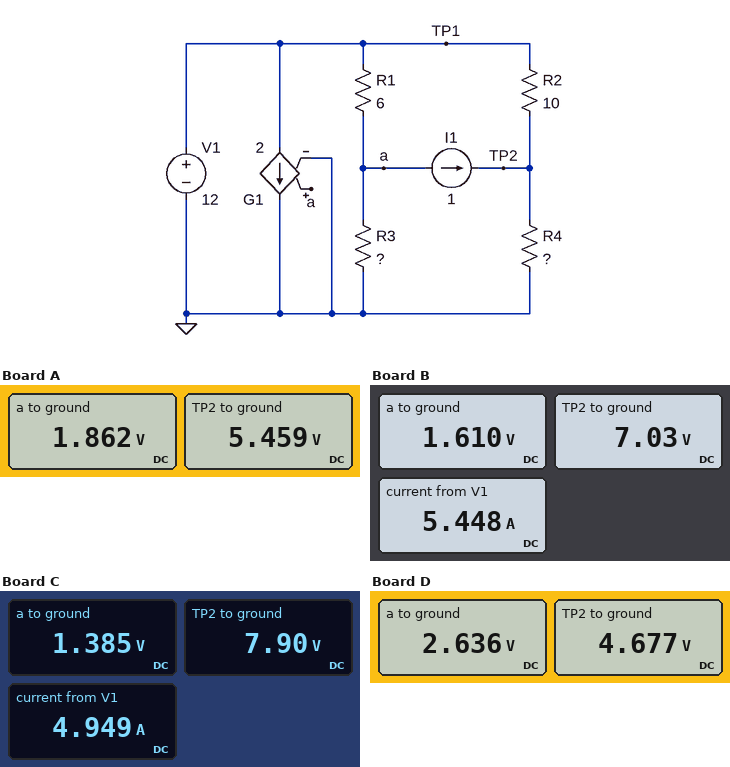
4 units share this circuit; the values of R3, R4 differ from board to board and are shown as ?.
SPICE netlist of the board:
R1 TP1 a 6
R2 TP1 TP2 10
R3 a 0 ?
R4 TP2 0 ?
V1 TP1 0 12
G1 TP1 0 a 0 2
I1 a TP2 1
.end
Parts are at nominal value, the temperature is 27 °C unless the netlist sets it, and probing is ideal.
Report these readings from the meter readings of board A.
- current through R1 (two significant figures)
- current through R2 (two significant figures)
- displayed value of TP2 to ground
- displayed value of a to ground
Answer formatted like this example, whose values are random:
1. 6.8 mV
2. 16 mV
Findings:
1. 1.7 A
2. 650 mA
3. 5.459 V
4. 1.862 V
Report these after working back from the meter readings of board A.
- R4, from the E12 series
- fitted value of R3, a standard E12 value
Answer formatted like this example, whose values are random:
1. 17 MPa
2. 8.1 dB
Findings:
1. 3.3 Ω
2. 2.7 Ω
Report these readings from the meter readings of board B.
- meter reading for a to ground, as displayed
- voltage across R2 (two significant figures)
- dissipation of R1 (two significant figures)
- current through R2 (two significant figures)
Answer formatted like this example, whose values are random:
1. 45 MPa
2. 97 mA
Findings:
1. 1.610 V
2. 5.0 V
3. 18 W
4. 500 mA
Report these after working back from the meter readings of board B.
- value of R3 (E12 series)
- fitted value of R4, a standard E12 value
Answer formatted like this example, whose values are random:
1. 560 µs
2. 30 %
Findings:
1. 2.2 Ω
2. 4.7 Ω
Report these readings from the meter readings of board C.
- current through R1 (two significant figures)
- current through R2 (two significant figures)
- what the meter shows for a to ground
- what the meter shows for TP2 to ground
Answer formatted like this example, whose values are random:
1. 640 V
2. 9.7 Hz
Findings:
1. 1.8 A
2. 410 mA
3. 1.385 V
4. 7.90 V
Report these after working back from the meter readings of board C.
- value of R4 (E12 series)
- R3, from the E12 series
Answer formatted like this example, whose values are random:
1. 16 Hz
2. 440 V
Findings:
1. 5.6 Ω
2. 1.8 Ω
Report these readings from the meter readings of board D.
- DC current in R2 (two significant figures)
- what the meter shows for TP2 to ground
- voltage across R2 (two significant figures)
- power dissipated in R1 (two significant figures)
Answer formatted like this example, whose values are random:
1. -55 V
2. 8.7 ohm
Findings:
1. 730 mA
2. 4.677 V
3. 7.3 V
4. 15 W
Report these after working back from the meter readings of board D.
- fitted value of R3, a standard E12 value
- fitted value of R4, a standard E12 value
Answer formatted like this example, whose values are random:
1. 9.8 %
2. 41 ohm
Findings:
1. 4.7 Ω
2. 2.7 Ω
